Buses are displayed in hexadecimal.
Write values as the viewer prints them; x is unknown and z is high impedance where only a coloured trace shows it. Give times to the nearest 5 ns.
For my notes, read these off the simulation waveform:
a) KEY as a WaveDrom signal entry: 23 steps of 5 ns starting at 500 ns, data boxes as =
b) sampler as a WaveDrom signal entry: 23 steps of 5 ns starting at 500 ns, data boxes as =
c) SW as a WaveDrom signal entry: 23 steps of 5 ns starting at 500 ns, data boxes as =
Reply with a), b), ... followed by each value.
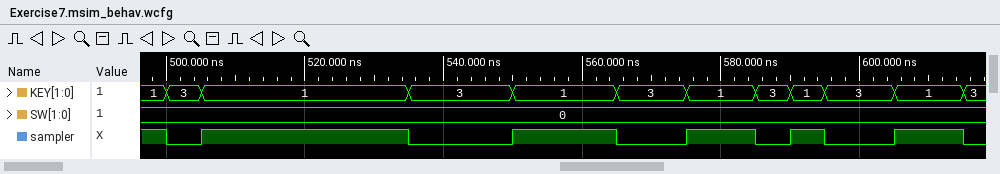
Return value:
a) {name: 'KEY', wave: '==.....=..=..=.=.===.=.', data: '3 1 3 1 3 1 3 1 3 1'}
b) {name: 'sampler', wave: '01.....0..1..0.1.010.1.'}
c) {name: 'SW', wave: '=......................', data: '0'}
